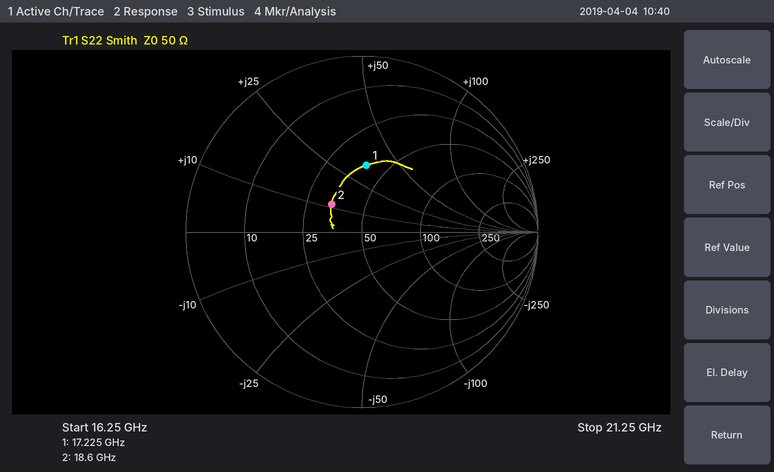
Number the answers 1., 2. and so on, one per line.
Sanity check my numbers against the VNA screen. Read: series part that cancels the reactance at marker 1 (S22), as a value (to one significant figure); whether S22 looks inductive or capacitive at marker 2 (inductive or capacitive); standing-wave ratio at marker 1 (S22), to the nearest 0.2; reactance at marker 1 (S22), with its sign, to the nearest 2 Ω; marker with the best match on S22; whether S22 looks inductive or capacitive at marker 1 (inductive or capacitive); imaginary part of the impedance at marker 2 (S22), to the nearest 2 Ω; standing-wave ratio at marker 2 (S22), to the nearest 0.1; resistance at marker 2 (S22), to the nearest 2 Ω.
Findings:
1. 300 fF
2. inductive
3. 2.2
4. +34 Ω
5. marker 2
6. inductive
7. +12 Ω
8. 1.6
9. 34 Ω
